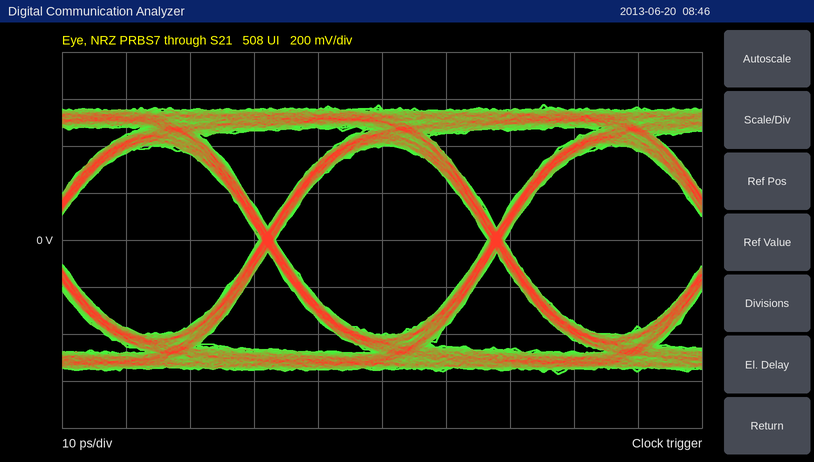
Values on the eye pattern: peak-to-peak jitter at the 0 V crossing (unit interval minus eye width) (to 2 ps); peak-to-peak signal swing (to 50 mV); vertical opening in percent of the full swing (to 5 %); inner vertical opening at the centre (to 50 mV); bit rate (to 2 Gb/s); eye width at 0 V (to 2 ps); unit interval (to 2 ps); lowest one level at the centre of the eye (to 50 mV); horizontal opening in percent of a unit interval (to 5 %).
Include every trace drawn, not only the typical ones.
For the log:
2 ps
1.15 V
70 %
800 mV
28 Gb/s
34 ps
36 ps
400 mV
95 %
